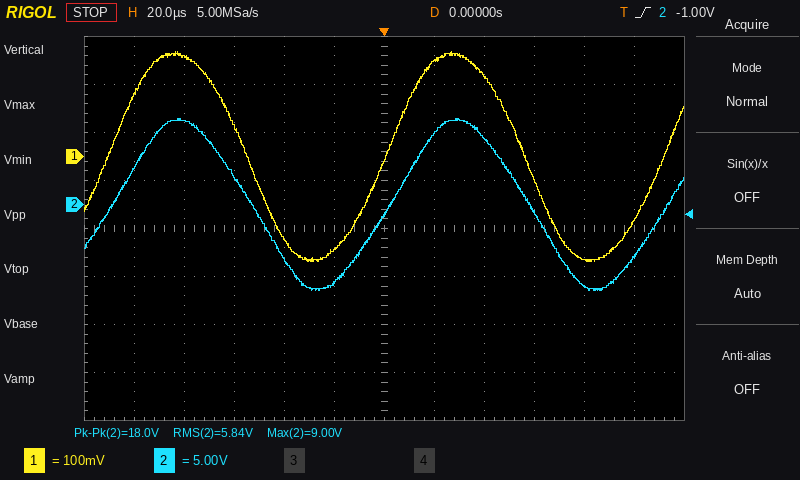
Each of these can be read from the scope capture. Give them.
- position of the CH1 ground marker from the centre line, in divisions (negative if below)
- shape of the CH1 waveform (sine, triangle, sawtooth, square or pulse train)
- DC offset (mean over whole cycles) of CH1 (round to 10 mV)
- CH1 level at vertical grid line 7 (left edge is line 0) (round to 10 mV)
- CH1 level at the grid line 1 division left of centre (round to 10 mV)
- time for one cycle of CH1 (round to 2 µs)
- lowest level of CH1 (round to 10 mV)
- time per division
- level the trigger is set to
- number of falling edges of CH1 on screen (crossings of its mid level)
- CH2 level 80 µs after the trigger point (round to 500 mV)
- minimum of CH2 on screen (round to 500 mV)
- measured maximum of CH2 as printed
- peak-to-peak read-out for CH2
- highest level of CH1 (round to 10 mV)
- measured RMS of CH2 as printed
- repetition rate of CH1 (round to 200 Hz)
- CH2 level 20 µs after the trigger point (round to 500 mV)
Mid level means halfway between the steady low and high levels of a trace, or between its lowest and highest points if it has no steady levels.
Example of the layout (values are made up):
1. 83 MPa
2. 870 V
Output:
1. +1.5 div
2. sine
3. 0 mV
4. 200 mV
5. -190 mV
6. 112 µs
7. -220 mV
8. 20 µs
9. -1.00 V
10. 2
11. -8.5 V
12. -9.0 V
13. 9.00 V
14. 18.0 V
15. 220 mV
16. 5.84 V
17. 9.0 kHz
18. 7.5 V
